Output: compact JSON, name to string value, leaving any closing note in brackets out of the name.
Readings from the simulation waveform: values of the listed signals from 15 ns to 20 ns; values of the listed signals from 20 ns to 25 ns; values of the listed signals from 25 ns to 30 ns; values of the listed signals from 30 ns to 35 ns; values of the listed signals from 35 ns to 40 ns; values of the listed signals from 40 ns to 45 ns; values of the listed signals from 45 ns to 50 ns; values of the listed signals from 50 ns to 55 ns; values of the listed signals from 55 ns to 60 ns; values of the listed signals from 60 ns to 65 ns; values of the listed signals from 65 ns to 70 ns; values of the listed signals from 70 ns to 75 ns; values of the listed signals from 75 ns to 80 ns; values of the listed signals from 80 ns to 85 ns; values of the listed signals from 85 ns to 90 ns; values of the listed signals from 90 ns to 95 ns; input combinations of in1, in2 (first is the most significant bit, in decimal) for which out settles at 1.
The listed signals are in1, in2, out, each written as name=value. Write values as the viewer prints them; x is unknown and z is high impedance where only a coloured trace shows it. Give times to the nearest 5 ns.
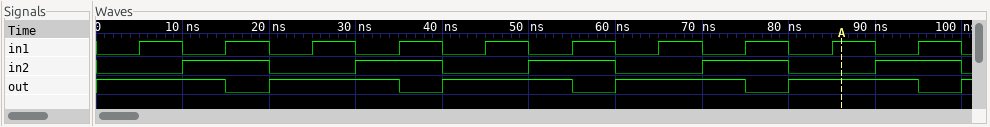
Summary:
{"values of the listed signals from 15 ns to 20 ns": "in1=1, in2=1, out=0", "values of the listed signals from 20 ns to 25 ns": "in1=0, in2=0, out=1", "values of the listed signals from 25 ns to 30 ns": "in1=1, in2=0, out=1", "values of the listed signals from 30 ns to 35 ns": "in1=0, in2=1, out=1", "values of the listed signals from 35 ns to 40 ns": "in1=1, in2=1, out=0", "values of the listed signals from 40 ns to 45 ns": "in1=0, in2=0, out=1", "values of the listed signals from 45 ns to 50 ns": "in1=1, in2=0, out=1", "values of the listed signals from 50 ns to 55 ns": "in1=0, in2=1, out=1", "values of the listed signals from 55 ns to 60 ns": "in1=1, in2=1, out=0", "values of the listed signals from 60 ns to 65 ns": "in1=0, in2=0, out=1", "values of the listed signals from 65 ns to 70 ns": "in1=1, in2=0, out=1", "values of the listed signals from 70 ns to 75 ns": "in1=0, in2=1, out=1", "values of the listed signals from 75 ns to 80 ns": "in1=1, in2=1, out=0", "values of the listed signals from 80 ns to 85 ns": "in1=0, in2=0, out=1", "values of the listed signals from 85 ns to 90 ns": "in1=1, in2=0, out=1", "values of the listed signals from 90 ns to 95 ns": "in1=0, in2=1, out=1", "input combinations of in1, in2 (first is the most significant bit, in decimal) for which out settles at 1": "0, 1, 2"}
